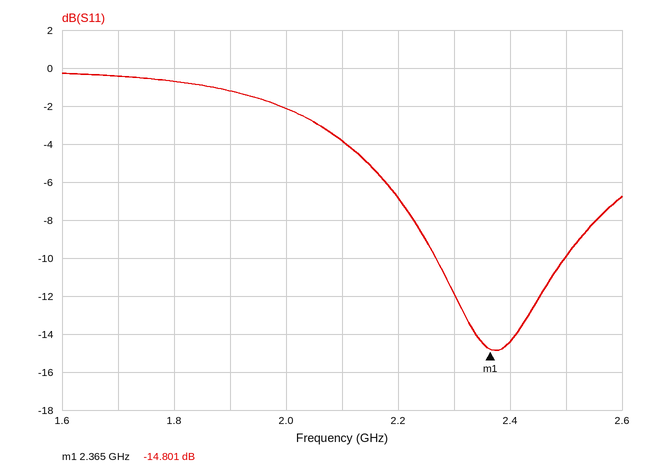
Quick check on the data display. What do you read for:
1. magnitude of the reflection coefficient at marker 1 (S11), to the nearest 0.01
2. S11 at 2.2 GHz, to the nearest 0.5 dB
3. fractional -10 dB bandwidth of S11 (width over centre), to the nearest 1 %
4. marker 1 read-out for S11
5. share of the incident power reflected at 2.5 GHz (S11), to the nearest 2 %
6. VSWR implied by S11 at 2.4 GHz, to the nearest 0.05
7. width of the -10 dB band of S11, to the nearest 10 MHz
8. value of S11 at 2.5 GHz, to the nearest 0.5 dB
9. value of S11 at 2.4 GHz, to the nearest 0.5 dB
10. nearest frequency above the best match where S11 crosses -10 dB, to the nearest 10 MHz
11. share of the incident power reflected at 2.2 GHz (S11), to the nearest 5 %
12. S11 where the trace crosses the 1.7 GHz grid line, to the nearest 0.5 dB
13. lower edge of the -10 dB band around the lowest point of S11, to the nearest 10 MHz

0.18
-7.0 dB
10 %
-14.801 dB
10 %
1.45
230 MHz
-10.0 dB
-14.5 dB
2.50 GHz
20 %
-0.5 dB
2.27 GHz
